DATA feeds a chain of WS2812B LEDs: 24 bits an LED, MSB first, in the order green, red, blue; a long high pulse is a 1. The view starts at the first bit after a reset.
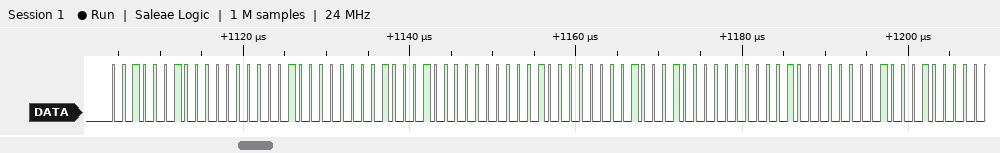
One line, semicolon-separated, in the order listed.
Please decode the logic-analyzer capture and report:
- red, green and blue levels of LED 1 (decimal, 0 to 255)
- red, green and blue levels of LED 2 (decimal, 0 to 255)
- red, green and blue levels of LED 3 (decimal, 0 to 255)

0, 34, 64; 0, 34, 64; 0, 34, 64
